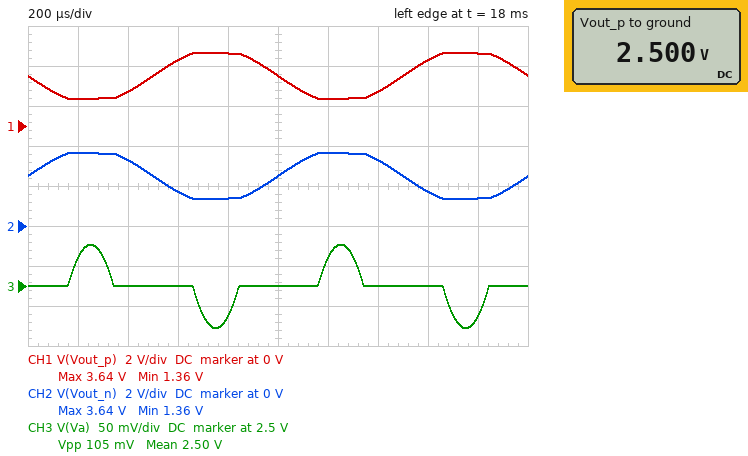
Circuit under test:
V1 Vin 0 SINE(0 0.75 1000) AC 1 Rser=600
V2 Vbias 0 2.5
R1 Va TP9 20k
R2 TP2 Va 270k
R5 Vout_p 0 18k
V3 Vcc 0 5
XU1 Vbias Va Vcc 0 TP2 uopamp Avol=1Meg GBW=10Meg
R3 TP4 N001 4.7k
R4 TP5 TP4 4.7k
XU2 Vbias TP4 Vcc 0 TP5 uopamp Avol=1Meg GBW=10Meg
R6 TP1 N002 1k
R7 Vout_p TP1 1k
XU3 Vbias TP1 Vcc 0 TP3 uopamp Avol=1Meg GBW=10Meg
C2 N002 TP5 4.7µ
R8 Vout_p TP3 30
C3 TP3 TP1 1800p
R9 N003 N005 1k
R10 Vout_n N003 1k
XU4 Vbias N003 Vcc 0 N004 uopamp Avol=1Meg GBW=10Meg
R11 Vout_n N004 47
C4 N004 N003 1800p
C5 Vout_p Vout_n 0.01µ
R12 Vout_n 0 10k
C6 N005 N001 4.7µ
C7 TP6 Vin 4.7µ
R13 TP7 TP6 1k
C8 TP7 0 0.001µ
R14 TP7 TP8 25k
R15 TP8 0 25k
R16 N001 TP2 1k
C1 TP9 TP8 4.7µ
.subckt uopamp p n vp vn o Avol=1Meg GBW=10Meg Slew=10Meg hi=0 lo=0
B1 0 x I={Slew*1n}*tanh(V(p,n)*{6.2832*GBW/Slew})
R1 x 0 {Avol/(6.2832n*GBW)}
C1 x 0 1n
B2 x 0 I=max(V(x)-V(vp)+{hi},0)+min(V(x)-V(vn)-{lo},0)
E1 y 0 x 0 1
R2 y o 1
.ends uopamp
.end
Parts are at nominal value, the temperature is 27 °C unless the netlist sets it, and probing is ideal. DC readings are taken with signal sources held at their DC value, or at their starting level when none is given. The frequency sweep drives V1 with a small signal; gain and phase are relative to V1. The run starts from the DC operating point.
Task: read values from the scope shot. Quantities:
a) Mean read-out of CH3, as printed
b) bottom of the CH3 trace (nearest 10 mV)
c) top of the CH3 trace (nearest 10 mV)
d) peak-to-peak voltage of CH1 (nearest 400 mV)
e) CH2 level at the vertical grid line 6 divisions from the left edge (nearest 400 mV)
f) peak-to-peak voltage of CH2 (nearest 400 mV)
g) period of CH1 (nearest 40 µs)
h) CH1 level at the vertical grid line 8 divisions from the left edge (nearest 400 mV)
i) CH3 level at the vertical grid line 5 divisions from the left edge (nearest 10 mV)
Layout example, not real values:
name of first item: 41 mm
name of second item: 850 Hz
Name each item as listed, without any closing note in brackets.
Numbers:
Mean read-out of CH3, as printed: 2.50 V
bottom of the CH3 trace: 2.45 V
top of the CH3 trace: 2.55 V
peak-to-peak voltage of CH1: 2.4 V
CH2 level at the vertical grid line 6 divisions from the left edge: 3.6 V
peak-to-peak voltage of CH2: 2.4 V
period of CH1: 1.00 ms
CH1 level at the vertical grid line 8 divisions from the left edge: 3.2 V
CH3 level at the vertical grid line 5 divisions from the left edge: 2.50 V
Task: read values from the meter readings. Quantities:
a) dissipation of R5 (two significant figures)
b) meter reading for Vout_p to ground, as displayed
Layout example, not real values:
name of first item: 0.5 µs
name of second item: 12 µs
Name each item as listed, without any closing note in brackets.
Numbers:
dissipation of R5: 350 µW
meter reading for Vout_p to ground, as displayed: 2.500 V
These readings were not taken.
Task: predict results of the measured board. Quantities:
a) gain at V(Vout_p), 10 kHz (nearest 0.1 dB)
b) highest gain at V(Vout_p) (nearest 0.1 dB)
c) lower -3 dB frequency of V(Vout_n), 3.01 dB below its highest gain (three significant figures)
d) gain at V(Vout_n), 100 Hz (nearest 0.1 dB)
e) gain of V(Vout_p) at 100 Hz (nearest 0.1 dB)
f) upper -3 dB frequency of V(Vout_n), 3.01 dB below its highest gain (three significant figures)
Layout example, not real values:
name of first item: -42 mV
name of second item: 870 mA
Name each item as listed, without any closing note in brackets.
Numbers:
gain at V(Vout_p), 10 kHz: 5.0 dB
highest gain at V(Vout_p): 5.1 dB
lower -3 dB frequency of V(Vout_n), 3.01 dB below its highest gain: 18.7 Hz
gain at V(Vout_n), 100 Hz: 4.9 dB
gain of V(Vout_p) at 100 Hz: 4.9 dB
upper -3 dB frequency of V(Vout_n), 3.01 dB below its highest gain: 81.2 kHz
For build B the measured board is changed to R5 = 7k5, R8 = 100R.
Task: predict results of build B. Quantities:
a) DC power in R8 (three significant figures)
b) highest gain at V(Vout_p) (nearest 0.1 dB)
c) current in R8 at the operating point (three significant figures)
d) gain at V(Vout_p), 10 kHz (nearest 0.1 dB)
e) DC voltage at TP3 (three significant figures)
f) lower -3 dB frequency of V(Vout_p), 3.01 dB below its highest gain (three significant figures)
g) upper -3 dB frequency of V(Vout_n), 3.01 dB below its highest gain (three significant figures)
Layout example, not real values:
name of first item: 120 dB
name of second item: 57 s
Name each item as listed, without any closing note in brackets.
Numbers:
DC power in R8: 11.1 µW
highest gain at V(Vout_p): 5.2 dB
current in R8 at the operating point: 333 µA
gain at V(Vout_p), 10 kHz: 5.1 dB
DC voltage at TP3: 2.53 V
lower -3 dB frequency of V(Vout_p), 3.01 dB below its highest gain: 19.1 Hz
upper -3 dB frequency of V(Vout_n), 3.01 dB below its highest gain: 77.0 kHz
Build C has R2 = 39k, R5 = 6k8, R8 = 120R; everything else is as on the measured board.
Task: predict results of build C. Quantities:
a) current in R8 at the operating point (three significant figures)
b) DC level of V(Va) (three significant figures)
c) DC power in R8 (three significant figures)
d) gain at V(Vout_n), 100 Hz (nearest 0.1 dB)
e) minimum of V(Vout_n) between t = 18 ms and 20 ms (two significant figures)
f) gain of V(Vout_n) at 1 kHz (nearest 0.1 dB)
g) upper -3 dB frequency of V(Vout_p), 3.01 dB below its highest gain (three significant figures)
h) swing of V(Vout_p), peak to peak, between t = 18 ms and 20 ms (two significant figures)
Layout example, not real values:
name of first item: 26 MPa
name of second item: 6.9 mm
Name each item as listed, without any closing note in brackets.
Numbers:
current in R8 at the operating point: 368 µA
DC level of V(Va): 2.50 V
DC power in R8: 16.2 µW
gain at V(Vout_n), 100 Hz: -11.9 dB
minimum of V(Vout_n) between t = 18 ms and 20 ms: 2.3 V
gain of V(Vout_n) at 1 kHz: -11.7 dB
upper -3 dB frequency of V(Vout_p), 3.01 dB below its highest gain: 95.7 kHz
swing of V(Vout_p), peak to peak, between t = 18 ms and 20 ms: 390 mV
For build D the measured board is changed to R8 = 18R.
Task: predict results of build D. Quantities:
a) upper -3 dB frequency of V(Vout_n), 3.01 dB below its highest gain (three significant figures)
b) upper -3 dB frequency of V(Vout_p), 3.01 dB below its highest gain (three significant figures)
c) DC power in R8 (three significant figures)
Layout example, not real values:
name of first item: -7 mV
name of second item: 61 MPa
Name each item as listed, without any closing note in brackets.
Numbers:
upper -3 dB frequency of V(Vout_n), 3.01 dB below its highest gain: 81.6 kHz
upper -3 dB frequency of V(Vout_p), 3.01 dB below its highest gain: 68.1 kHz
DC power in R8: 347 nW
